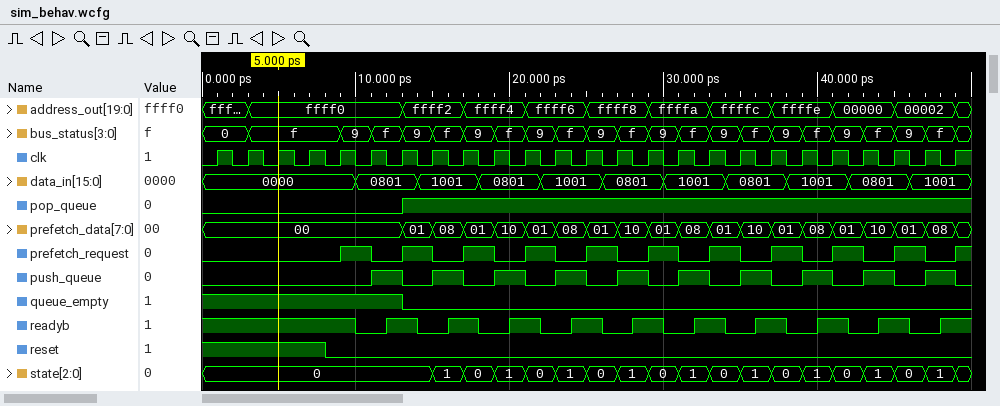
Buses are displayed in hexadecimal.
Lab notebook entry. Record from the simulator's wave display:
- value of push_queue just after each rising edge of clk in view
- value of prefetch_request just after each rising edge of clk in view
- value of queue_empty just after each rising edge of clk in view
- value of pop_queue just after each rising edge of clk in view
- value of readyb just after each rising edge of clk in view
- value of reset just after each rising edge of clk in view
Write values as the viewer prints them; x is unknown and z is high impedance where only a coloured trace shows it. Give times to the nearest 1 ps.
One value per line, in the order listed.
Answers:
0 0 0 0 0 1 0 1 0 1 0 1 0 1 0 1 0 1 0 1 0 1 0 1 0
0 0 0 0 1 0 1 0 1 0 1 0 1 0 1 0 1 0 1 0 1 0 1 0 1
1 1 1 1 1 1 0 0 0 0 0 0 0 0 0 0 0 0 0 0 0 0 0 0 0
0 0 0 0 0 0 1 1 1 1 1 1 1 1 1 1 1 1 1 1 1 1 1 1 1
1 1 1 1 1 0 1 0 1 0 1 0 1 0 1 0 1 0 1 0 1 0 1 0 1
1 1 1 1 0 0 0 0 0 0 0 0 0 0 0 0 0 0 0 0 0 0 0 0 0
